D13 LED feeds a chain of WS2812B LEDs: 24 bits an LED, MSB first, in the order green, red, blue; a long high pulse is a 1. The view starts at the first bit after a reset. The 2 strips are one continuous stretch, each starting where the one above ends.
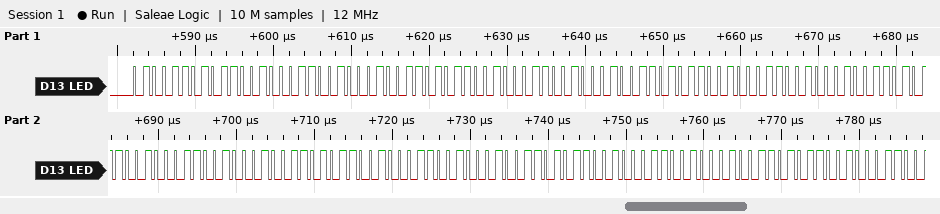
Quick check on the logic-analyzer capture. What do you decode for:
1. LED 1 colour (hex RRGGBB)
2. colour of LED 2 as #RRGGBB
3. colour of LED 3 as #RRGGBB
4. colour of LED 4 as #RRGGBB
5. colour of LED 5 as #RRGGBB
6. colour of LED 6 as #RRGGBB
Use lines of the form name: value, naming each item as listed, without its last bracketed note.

LED 1 colour: #644D64
colour of LED 2 as #RRGGBB: #644D64
colour of LED 3 as #RRGGBB: #644D64
colour of LED 4 as #RRGGBB: #644D64
colour of LED 5 as #RRGGBB: #644D64
colour of LED 6 as #RRGGBB: #644D64
